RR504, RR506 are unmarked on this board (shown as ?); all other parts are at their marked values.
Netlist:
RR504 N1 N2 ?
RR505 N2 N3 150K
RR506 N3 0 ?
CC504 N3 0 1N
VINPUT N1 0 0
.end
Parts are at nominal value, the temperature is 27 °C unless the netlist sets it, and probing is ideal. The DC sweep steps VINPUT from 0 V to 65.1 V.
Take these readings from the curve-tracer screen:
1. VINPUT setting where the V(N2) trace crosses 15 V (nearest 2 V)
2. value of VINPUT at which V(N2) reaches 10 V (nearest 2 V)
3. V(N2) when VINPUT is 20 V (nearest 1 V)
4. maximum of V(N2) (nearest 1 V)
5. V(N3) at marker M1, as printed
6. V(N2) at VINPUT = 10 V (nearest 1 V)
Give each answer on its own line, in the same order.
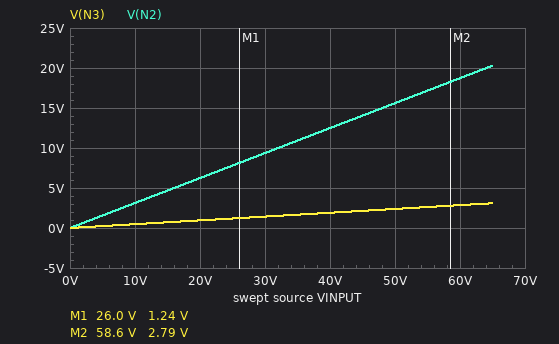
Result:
48 V
32 V
6 V
20 V
1.24 V
3 V
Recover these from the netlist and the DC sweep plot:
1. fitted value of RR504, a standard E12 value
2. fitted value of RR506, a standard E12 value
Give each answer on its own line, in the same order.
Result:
390 kΩ
27 kΩ
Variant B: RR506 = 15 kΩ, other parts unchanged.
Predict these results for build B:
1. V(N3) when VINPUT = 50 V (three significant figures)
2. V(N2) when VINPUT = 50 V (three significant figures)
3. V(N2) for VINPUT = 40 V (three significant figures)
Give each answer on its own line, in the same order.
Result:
1.35 V
14.9 V
11.9 V
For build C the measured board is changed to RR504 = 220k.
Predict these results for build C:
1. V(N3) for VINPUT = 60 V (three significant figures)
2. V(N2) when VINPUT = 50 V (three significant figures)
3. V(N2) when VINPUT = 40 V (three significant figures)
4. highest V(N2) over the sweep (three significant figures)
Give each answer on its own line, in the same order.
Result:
4.08 V
22.3 V
17.8 V
29.0 V
